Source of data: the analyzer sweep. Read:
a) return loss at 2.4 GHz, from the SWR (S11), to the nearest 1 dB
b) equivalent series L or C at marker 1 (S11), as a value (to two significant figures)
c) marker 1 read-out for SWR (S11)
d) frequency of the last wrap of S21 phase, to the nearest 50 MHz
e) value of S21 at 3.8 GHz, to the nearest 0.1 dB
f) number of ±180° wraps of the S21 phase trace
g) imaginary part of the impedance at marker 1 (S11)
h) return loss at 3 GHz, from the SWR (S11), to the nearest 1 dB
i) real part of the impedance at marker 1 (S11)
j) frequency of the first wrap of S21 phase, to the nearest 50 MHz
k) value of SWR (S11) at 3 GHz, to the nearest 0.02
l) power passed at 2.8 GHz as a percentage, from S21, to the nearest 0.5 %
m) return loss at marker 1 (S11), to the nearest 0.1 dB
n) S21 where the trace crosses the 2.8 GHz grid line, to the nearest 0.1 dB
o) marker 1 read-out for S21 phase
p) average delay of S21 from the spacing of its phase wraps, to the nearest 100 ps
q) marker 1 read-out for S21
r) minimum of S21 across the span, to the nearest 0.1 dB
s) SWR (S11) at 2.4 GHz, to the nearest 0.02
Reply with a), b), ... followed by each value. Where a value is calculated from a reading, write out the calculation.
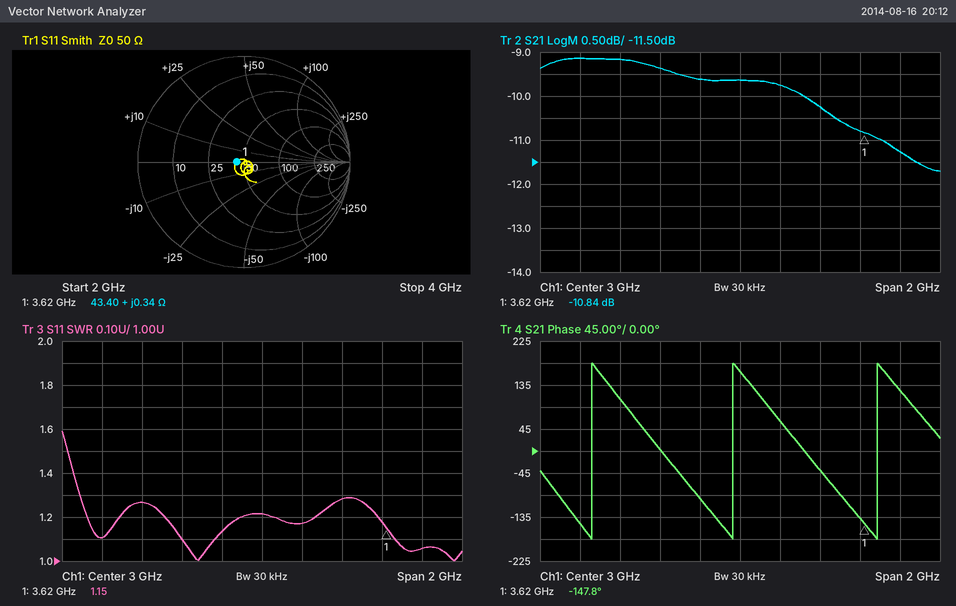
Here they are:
a) −20 log10((1.26 − 1)/(1.26 + 1)) ≈ 19 dB
b) L = 0.34 Ω/(2π × 3.62 GHz) ≈ 15 pH
c) 1.15
d) 3.70 GHz
e) -11.3 dB
f) 3
g) +0.34 Ω
h) −20 log10((1.22 − 1)/(1.22 + 1)) ≈ 20 dB
i) 43.40 Ω
j) 2.25 GHz
k) 1.22
l) 10^(-9.6/10) ≈ 11.0 %
m) 23.0 dB
n) -9.6 dB
o) -147.8°
p) 2 cycles / (3.70 GHz − 2.25 GHz) ≈ 1.4 ns
q) -10.84 dB
r) -11.7 dB
s) 1.26
